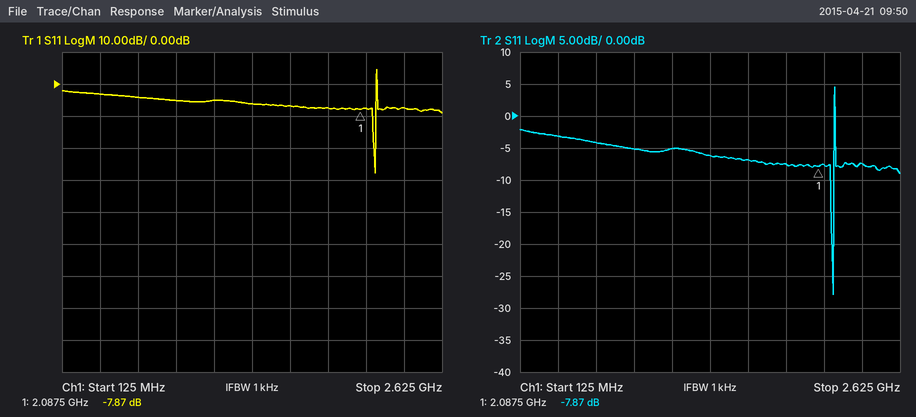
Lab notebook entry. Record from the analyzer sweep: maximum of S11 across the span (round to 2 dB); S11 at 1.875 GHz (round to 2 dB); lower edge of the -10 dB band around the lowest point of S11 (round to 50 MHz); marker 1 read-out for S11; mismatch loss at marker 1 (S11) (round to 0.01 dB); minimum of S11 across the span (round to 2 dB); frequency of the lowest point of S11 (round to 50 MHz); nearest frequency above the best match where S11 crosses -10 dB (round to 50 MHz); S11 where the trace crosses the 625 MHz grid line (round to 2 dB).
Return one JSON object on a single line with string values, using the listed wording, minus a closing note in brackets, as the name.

{"maximum of S11 across the span": "4 dB", "S11 at 1.875 GHz": "-8 dB", "lower edge of the -10 dB band around the lowest point of S11": "2.15 GHz", "marker 1 read-out for S11": "-7.87 dB", "mismatch loss at marker 1 (S11)": "0.77 dB", "minimum of S11 across the span": "-28 dB", "frequency of the lowest point of S11": "2.20 GHz", "nearest frequency above the best match where S11 crosses -10 dB": "2.20 GHz", "S11 where the trace crosses the 625 MHz grid line": "-4 dB"}
